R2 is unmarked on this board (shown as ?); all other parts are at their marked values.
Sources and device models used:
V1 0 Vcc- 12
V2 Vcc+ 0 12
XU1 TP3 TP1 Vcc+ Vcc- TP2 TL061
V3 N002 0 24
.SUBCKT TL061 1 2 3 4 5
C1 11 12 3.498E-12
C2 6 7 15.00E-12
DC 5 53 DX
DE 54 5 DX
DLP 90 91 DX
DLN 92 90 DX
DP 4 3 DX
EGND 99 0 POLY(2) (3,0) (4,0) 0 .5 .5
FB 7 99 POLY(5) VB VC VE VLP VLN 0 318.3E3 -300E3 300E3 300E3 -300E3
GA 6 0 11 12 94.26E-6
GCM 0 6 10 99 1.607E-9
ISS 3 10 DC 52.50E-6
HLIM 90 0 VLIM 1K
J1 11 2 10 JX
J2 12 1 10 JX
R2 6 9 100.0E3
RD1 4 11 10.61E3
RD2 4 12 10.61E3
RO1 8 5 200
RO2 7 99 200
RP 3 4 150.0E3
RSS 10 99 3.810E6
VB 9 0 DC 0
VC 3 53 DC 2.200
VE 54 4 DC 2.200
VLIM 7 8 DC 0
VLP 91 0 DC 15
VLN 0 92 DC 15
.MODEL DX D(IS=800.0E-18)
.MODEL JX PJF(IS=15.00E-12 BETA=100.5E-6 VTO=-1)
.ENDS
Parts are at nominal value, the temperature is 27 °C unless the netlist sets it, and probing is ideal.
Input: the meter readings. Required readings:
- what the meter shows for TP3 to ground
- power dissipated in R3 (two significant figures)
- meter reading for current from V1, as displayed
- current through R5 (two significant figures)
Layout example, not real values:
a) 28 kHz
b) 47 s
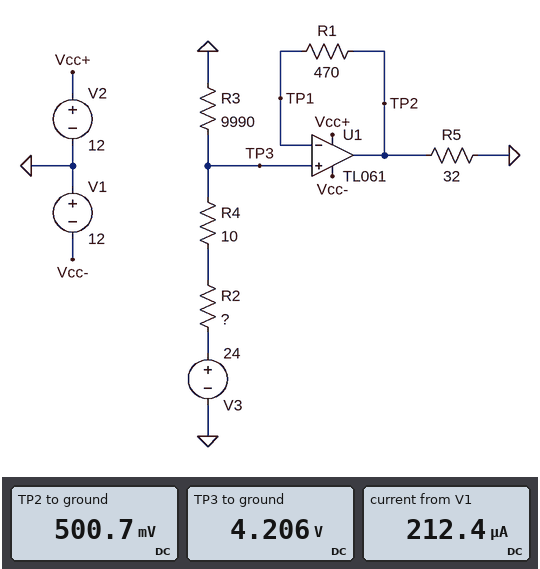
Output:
a) 4.206 V
b) 1.8 mW
c) 212.4 µA
d) 16 mA
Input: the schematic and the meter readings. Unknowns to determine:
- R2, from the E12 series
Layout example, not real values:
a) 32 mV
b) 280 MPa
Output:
a) 47 kΩ
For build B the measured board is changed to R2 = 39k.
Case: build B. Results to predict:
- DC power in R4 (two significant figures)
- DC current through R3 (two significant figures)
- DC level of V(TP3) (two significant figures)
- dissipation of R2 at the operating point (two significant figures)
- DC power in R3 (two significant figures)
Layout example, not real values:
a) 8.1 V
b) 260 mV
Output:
a) 2.4 µW
b) 490 µA
c) 4.9 V
d) 9.4 mW
e) 2.4 mW
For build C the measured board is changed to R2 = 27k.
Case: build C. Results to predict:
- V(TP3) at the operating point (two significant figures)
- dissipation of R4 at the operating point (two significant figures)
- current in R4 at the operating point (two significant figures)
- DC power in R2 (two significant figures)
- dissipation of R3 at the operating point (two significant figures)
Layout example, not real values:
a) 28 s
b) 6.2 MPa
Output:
a) 6.5 V
b) 4.2 µW
c) 650 µA
d) 11 mW
e) 4.2 mW
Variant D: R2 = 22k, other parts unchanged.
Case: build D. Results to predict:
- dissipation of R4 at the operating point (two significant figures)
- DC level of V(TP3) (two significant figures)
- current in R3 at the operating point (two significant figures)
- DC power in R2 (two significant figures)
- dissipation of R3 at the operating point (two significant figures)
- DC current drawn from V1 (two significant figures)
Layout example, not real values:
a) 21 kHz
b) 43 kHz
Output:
a) 5.6 µW
b) 7.5 V
c) 750 µA
d) 12 mW
e) 5.6 mW
f) 210 µA
